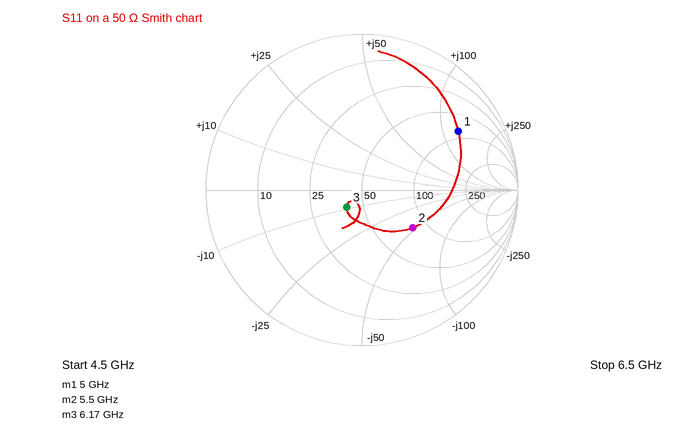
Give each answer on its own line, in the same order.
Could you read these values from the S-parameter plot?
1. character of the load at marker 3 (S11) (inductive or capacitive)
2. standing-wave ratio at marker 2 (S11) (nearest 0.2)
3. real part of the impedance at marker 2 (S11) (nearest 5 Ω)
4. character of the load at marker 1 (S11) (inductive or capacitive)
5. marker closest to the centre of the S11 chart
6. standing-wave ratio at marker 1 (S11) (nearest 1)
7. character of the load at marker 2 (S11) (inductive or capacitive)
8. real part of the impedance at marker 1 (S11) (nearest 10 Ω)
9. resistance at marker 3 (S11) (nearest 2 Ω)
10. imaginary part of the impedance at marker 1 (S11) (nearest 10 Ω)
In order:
capacitive
2.4
80 Ω
inductive
marker 3
6
capacitive
80 Ω
40 Ω
+130 Ω
